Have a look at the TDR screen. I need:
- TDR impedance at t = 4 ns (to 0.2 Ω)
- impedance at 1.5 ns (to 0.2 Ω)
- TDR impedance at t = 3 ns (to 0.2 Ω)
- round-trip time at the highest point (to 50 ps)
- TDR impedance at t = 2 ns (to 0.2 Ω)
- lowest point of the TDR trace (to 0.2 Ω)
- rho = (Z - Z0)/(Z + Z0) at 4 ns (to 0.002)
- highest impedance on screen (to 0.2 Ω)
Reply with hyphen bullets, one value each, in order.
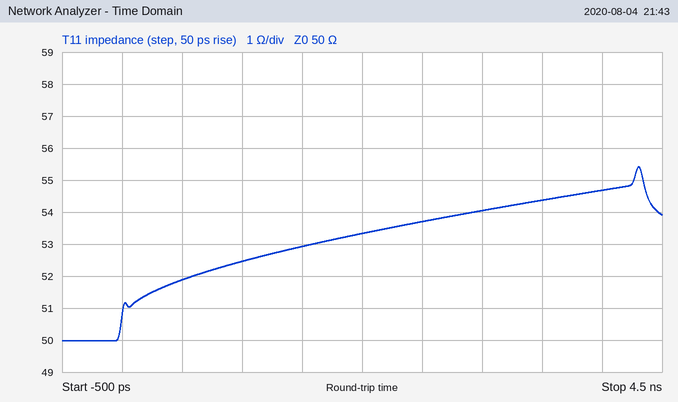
- 54.6 Ω
- 53.0 Ω
- 54.0 Ω
- 4.30 ns
- 53.4 Ω
- 50.0 Ω
- +0.044
- 55.4 Ω
